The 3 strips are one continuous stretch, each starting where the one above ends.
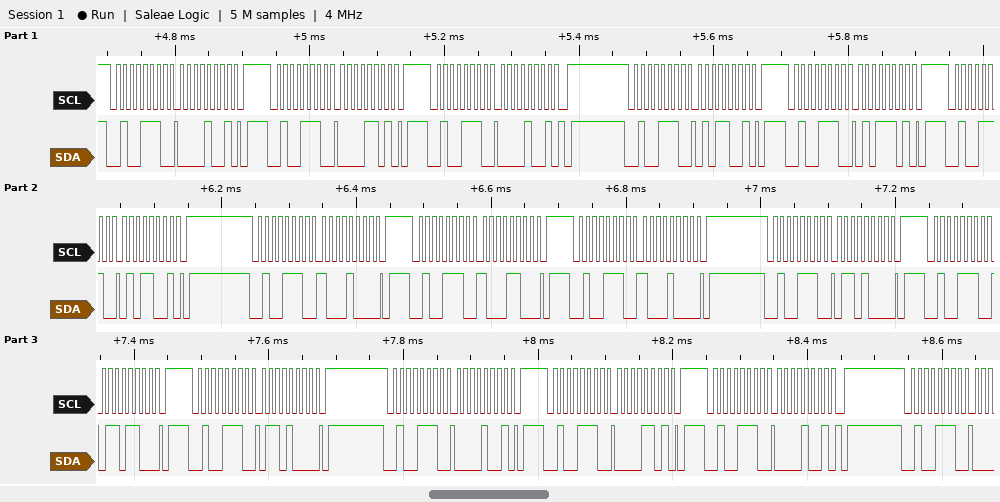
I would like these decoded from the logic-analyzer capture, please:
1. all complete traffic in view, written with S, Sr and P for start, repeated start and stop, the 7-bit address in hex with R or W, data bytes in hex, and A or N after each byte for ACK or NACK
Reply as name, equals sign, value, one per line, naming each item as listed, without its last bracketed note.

all complete traffic in view, written with S, Sr and P for start, repeated start and stop, the 7-bit address in hex with R or W, data bytes in hex, and A or N after each byte for ACK or NACK = S 27W A 09 A P S 27W A 0D A P S 27W A 09 A P S 27W A 59 A P S 27W A 5D A P S 27W A 59 A P S 27W A 88 A P S 27W A 8C A P S 27W A 88 A P S 27W A 68 A P S 27W A 6C A P S 27W A 68 A P S 27W A 09 A P S 27W A 0D A P S 27W A 09 A P S 27W A
